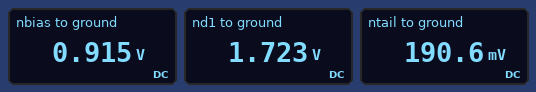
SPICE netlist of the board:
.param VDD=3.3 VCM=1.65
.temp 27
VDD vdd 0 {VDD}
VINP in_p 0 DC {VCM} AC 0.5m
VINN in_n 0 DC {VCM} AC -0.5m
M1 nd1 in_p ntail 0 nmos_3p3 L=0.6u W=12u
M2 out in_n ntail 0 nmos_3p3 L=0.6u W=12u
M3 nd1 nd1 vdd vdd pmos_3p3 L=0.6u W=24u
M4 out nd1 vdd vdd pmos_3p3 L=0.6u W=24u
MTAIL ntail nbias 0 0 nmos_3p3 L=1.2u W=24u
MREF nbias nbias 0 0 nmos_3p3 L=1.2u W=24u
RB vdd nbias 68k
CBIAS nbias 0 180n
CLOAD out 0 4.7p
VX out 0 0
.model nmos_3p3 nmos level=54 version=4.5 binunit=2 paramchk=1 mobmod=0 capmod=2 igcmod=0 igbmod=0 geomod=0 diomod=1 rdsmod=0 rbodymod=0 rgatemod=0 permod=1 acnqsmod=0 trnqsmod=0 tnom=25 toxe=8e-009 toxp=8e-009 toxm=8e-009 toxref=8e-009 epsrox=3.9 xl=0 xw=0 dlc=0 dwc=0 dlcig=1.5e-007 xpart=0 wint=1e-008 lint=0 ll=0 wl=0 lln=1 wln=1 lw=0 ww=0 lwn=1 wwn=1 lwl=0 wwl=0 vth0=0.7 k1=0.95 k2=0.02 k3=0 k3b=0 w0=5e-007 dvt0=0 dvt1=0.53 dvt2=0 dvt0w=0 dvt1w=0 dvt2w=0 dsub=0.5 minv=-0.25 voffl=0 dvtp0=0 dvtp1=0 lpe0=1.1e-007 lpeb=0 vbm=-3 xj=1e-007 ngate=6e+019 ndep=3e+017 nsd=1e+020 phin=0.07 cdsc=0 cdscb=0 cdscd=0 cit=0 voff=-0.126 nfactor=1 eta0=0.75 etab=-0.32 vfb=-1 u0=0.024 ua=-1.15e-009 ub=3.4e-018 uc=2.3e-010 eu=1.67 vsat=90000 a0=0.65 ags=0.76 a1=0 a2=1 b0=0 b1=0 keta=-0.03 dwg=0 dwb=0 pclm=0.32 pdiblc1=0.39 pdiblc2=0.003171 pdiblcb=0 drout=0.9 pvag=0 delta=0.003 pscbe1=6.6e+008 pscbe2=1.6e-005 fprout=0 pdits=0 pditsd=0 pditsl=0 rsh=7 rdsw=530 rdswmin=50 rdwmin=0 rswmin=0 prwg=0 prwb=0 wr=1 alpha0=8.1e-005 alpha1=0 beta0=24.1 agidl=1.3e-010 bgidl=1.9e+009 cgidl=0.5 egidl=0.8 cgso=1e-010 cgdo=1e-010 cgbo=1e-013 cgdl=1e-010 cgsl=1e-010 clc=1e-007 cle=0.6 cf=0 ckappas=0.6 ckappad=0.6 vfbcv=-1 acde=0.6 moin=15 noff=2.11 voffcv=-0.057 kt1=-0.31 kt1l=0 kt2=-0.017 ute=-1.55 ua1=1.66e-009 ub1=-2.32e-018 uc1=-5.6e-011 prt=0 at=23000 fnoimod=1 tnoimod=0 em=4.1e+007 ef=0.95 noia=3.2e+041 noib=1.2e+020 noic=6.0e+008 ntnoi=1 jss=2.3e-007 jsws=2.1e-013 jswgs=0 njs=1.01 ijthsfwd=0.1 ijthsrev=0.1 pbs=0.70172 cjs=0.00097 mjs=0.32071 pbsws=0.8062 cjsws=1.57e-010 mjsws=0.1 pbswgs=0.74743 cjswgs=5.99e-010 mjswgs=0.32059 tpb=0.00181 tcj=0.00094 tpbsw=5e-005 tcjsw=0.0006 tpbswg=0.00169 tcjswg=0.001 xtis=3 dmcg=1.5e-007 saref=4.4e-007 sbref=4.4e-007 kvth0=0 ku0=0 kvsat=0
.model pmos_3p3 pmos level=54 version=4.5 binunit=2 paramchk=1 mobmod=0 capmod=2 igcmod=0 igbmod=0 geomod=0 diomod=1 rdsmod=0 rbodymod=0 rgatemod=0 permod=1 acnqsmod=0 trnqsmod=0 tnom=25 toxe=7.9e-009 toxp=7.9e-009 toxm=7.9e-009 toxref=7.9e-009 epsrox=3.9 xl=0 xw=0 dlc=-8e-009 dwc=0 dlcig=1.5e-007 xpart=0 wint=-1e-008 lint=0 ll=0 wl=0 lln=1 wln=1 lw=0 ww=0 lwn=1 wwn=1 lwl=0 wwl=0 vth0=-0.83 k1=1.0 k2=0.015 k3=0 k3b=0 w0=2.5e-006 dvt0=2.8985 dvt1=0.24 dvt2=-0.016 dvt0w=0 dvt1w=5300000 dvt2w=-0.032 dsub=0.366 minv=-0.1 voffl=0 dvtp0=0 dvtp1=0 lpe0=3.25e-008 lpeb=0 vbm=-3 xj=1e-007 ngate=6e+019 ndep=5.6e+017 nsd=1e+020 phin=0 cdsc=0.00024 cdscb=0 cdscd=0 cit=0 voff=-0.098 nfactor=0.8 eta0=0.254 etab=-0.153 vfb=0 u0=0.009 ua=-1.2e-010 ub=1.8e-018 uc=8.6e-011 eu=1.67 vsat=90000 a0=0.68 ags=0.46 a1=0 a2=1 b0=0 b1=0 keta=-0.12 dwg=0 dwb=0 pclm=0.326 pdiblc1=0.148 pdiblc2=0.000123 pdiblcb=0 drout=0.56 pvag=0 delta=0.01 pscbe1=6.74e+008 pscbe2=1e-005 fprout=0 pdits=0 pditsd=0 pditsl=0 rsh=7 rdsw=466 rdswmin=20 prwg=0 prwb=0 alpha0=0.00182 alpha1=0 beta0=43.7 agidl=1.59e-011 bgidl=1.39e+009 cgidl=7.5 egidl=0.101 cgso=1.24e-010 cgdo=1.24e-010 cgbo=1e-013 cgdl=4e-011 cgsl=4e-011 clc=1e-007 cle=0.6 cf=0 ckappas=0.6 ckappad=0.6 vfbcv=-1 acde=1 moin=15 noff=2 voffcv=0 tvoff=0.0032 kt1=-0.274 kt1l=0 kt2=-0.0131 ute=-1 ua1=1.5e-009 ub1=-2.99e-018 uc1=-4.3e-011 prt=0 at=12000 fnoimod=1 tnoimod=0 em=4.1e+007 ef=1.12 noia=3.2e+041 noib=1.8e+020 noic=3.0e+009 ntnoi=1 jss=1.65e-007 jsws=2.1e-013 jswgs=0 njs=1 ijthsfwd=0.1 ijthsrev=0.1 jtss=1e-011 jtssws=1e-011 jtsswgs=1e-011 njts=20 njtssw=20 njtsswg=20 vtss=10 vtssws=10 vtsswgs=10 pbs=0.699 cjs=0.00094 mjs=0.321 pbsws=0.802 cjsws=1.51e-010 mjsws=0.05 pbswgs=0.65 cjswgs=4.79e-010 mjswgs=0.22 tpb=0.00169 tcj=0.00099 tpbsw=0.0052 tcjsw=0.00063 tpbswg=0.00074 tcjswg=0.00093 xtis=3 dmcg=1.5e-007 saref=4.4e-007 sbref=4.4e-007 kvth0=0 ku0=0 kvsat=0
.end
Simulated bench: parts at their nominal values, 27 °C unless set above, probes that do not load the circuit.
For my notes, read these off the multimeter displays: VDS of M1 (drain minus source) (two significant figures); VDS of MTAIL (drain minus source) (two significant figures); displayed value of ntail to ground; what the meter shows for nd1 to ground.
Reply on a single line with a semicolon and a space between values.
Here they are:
1.5 V; 190 mV; 190.6 mV; 1.723 V
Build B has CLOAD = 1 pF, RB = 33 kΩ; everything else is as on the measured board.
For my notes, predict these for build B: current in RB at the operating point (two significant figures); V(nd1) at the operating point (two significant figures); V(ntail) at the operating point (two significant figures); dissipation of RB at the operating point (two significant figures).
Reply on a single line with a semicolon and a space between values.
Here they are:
70 µA; 1.7 V; 180 mV; 160 µW
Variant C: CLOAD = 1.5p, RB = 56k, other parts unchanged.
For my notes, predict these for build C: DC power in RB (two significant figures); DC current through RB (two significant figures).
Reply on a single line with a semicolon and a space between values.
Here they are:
100 µW; 42 µA
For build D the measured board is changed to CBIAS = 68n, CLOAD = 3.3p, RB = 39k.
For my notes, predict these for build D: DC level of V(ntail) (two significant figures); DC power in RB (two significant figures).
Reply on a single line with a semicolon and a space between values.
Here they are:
180 mV; 140 µW
